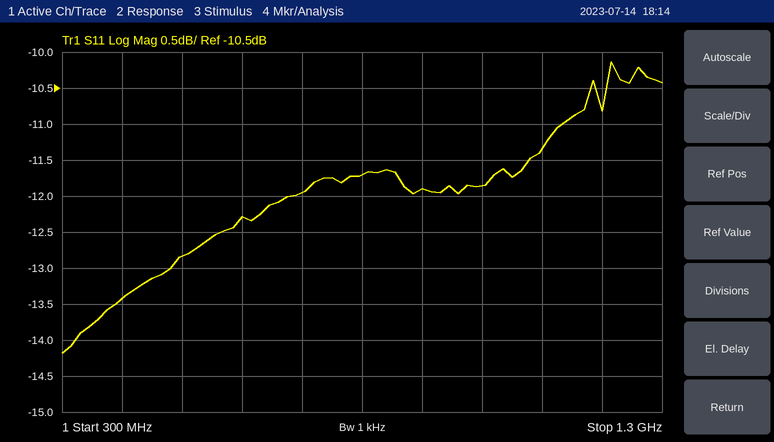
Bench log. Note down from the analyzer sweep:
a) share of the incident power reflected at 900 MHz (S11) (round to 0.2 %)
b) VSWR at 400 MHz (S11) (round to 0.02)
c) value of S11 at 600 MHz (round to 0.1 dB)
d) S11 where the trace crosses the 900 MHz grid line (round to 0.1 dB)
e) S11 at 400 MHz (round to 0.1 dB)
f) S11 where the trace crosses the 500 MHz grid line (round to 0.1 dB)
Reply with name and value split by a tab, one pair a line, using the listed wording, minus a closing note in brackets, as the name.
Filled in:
share of the incident power reflected at 900 MHz (S11)	6.4 %
VSWR at 400 MHz (S11)	1.54
value of S11 at 600 MHz	-12.3 dB
S11 where the trace crosses the 900 MHz grid line	-11.9 dB
S11 at 400 MHz	-13.4 dB
S11 where the trace crosses the 500 MHz grid line	-12.8 dB
